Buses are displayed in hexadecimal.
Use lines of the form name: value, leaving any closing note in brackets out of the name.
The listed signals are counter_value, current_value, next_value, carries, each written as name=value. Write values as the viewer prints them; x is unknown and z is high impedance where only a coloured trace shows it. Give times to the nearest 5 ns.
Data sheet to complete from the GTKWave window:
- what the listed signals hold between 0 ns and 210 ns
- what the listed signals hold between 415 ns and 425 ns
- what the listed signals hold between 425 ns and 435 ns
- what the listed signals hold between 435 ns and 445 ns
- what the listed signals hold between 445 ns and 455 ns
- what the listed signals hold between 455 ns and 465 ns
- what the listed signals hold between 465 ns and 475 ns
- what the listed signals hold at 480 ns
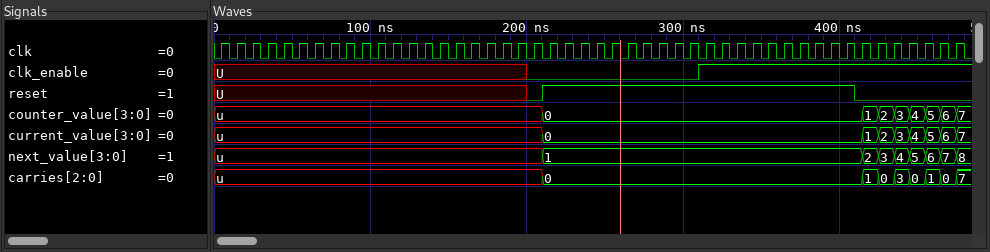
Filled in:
what the listed signals hold between 0 ns and 210 ns: counter_value=u, current_value=u, next_value=u, carries=u
what the listed signals hold between 415 ns and 425 ns: counter_value=1, current_value=1, next_value=2, carries=1
what the listed signals hold between 425 ns and 435 ns: counter_value=2, current_value=2, next_value=3, carries=0
what the listed signals hold between 435 ns and 445 ns: counter_value=3, current_value=3, next_value=4, carries=3
what the listed signals hold between 445 ns and 455 ns: counter_value=4, current_value=4, next_value=5, carries=0
what the listed signals hold between 455 ns and 465 ns: counter_value=5, current_value=5, next_value=6, carries=1
what the listed signals hold between 465 ns and 475 ns: counter_value=6, current_value=6, next_value=7, carries=0
what the listed signals hold at 480 ns: counter_value=7, current_value=7, next_value=8, carries=7
